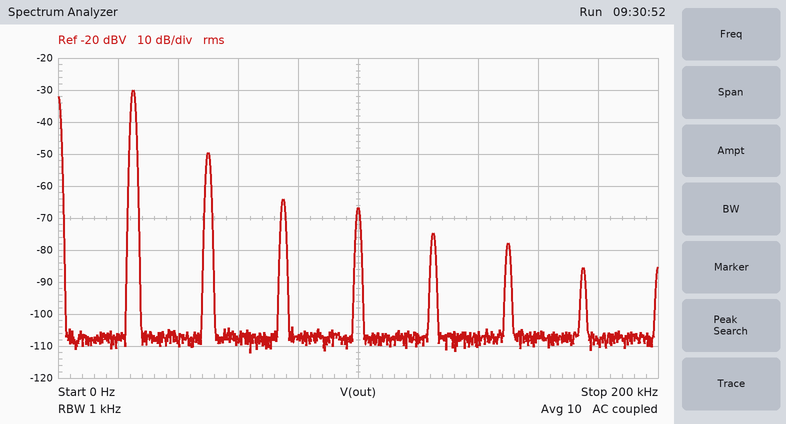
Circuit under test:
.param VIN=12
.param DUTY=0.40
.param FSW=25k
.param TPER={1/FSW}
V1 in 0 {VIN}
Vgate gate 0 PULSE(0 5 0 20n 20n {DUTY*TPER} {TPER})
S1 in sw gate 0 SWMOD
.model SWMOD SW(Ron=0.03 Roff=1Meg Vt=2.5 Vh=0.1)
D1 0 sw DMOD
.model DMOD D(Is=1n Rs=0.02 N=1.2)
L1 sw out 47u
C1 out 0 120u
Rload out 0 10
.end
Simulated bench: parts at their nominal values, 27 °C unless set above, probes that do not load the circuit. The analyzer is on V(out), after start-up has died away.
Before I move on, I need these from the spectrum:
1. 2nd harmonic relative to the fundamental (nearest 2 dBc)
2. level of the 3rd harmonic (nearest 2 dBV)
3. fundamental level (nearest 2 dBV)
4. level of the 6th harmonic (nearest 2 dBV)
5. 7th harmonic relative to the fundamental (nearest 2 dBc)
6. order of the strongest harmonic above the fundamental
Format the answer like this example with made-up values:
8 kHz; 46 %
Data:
-20 dBc; -64 dBV; -30 dBV; -78 dBV; -56 dBc; 2
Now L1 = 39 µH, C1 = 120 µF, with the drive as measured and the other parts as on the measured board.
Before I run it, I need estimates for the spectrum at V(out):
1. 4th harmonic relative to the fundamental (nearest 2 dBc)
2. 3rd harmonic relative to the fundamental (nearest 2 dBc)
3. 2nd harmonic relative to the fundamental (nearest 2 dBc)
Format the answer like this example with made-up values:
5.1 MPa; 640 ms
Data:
-40 dBc; -30 dBc; -18 dBc
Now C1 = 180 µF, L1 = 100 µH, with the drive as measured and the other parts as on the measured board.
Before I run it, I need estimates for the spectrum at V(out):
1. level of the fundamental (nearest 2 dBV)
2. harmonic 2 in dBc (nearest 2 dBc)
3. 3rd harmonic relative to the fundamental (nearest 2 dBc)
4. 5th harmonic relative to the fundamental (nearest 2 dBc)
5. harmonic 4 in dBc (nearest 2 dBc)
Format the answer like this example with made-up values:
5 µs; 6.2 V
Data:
-38 dBV; -28 dBc; -32 dBc; -48 dBc; -42 dBc
